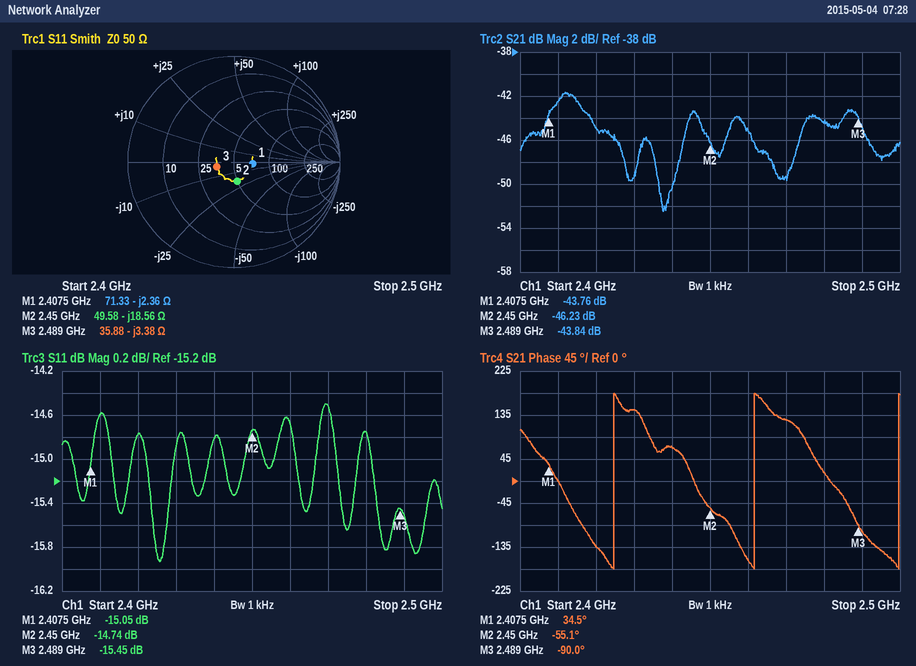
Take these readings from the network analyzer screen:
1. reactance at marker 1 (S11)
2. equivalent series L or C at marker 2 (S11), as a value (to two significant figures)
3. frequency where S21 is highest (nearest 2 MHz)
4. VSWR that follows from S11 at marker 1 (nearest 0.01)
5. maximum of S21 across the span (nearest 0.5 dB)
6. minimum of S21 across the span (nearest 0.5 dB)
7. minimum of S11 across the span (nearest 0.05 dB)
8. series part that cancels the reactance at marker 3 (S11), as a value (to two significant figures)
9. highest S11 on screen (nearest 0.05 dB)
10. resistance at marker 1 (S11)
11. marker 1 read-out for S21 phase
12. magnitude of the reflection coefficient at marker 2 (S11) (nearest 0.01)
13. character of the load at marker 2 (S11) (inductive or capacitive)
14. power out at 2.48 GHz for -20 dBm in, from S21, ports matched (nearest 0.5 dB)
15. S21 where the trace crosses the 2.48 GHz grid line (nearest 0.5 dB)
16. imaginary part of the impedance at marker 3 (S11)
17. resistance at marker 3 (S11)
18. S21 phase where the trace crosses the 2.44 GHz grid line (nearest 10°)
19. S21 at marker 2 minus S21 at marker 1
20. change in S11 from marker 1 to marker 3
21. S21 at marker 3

-2.36 Ω
3.5 pF
2.412 GHz
1.43
-41.5 dB
-52.5 dB
-15.95 dB
220 pH
-14.50 dB
71.33 Ω
34.5°
0.18
capacitive
-64.5 dBm
-44.5 dB
-3.38 Ω
35.88 Ω
70°
-2.47 dB
-0.40 dB
-43.84 dB
